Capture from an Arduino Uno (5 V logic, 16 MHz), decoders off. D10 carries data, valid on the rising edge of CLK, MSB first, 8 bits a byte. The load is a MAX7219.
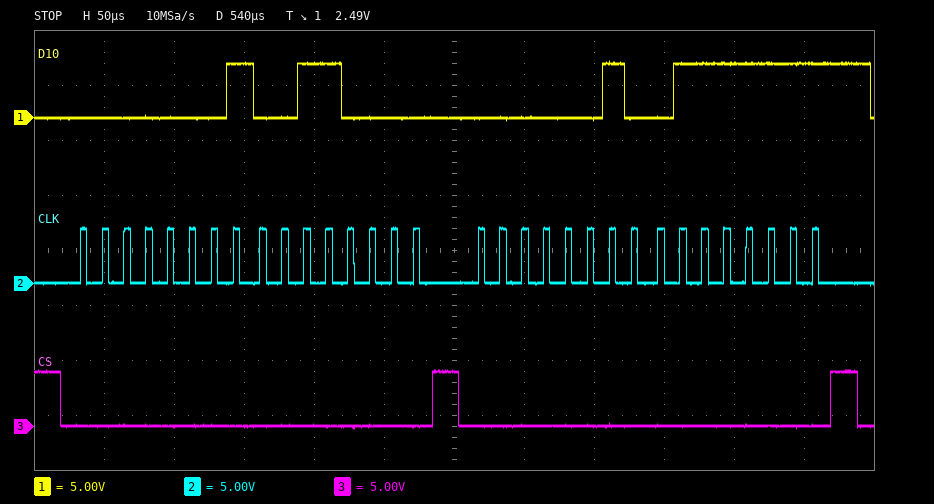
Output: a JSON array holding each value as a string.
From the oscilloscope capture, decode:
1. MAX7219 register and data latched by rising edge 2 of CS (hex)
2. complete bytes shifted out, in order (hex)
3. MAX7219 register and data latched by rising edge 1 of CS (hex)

["register 0x2, data 0x7F", "01 30 02 7F", "register 0x1, data 0x30"]
